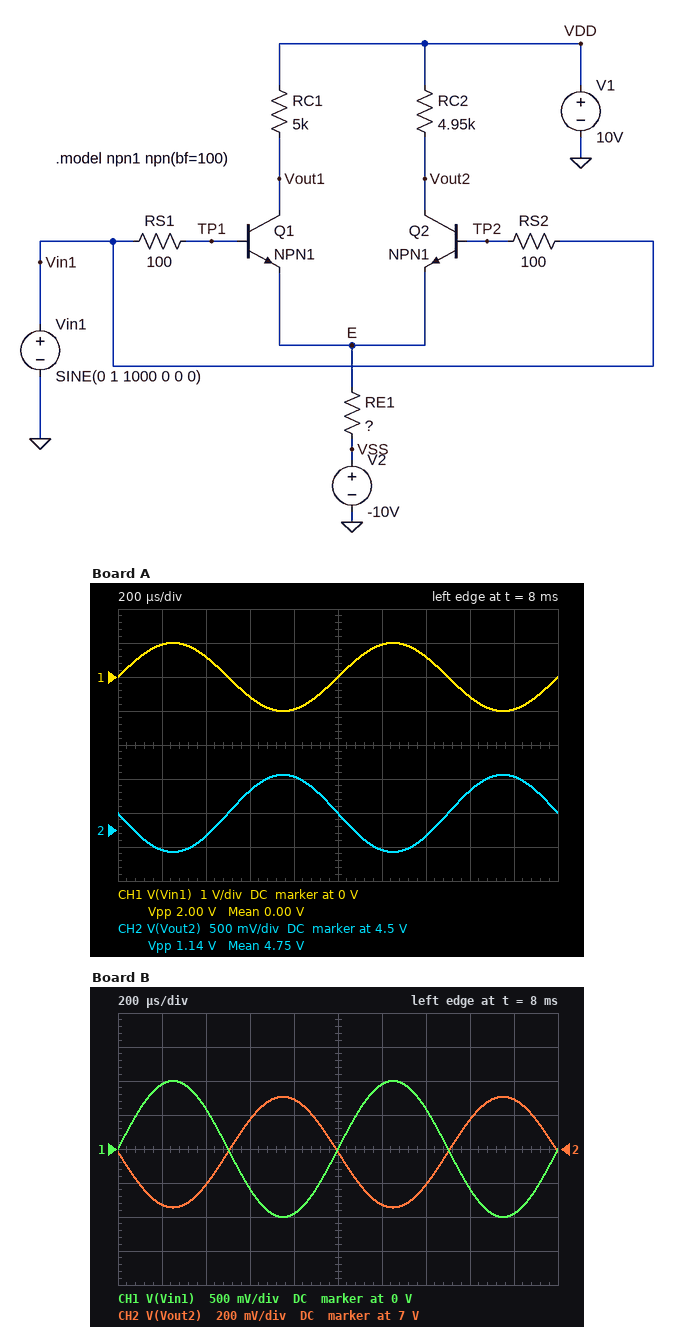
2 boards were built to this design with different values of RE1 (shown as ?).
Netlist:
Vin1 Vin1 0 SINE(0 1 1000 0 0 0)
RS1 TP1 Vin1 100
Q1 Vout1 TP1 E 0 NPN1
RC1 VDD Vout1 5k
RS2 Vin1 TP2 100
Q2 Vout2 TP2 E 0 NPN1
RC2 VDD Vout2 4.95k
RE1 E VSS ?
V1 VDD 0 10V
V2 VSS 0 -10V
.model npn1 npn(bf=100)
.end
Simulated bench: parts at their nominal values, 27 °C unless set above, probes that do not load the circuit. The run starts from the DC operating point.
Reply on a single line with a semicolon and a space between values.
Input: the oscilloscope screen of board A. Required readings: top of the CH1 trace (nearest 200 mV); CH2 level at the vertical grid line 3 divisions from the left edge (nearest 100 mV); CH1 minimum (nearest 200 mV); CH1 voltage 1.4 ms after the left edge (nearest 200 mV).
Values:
1.0 V; 5.1 V; -1.0 V; 600 mV
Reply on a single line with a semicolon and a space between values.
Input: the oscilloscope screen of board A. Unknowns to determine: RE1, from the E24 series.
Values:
4.3 kΩ
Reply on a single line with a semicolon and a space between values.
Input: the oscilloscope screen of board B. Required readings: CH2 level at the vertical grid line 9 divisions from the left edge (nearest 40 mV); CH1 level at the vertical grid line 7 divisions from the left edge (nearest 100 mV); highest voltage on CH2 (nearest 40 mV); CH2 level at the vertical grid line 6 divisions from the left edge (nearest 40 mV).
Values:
7.28 V; 600 mV; 7.32 V; 6.68 V
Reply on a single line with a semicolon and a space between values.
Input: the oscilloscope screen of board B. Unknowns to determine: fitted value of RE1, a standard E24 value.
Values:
7.5 kΩ
